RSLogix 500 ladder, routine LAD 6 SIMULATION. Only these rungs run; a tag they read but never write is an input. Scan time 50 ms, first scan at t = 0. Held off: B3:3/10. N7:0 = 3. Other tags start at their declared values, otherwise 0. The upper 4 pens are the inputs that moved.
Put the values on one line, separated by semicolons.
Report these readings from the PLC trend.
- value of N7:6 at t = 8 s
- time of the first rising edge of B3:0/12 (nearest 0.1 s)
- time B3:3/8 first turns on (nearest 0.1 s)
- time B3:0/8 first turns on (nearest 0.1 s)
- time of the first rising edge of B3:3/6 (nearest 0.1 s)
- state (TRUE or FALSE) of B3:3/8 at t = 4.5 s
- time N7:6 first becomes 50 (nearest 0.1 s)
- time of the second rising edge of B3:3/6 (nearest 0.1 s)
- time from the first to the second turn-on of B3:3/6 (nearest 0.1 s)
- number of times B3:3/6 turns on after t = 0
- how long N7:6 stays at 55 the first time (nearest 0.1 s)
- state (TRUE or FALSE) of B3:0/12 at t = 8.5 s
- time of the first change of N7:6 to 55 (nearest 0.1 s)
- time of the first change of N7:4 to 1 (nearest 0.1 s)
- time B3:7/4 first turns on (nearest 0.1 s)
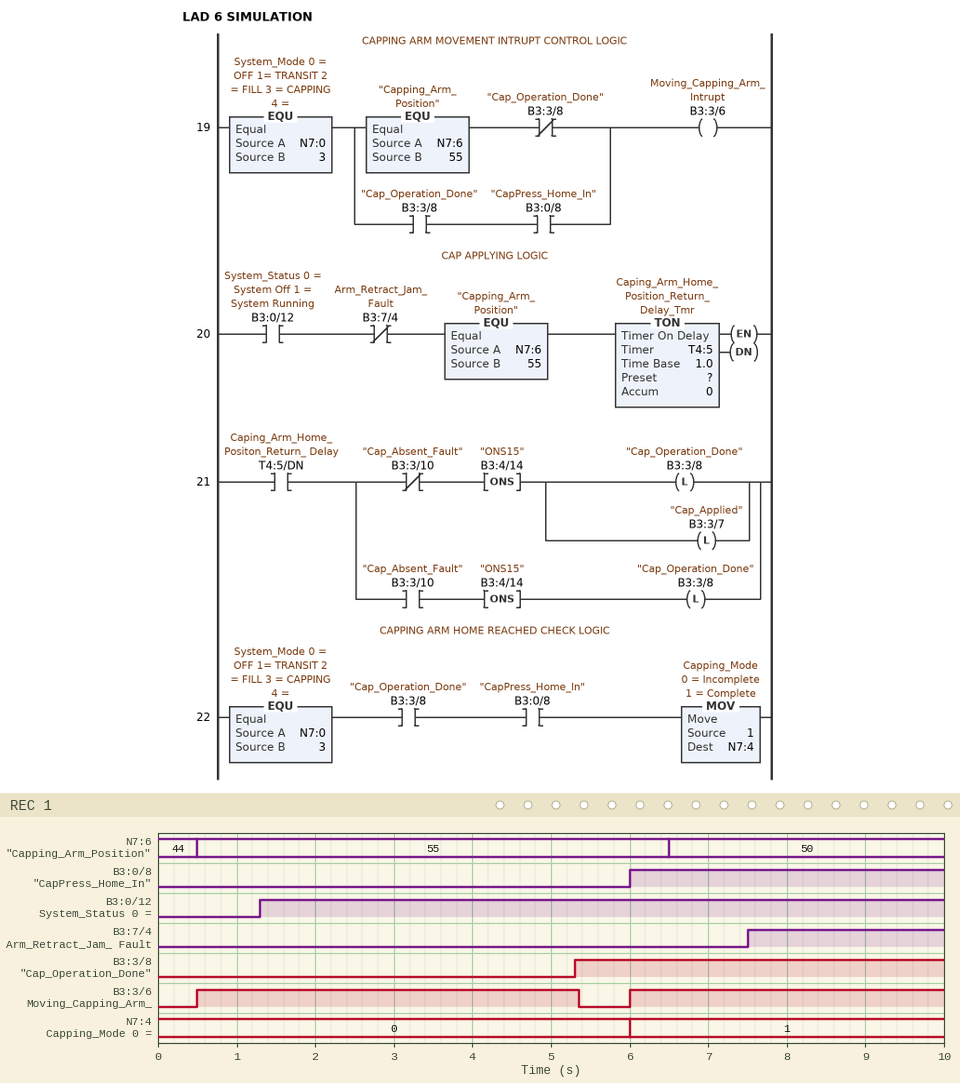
50; 1.3 s; 5.3 s; 6.0 s; 0.5 s; FALSE; 6.5 s; 6.0 s; 5.5 s; 2; 6.0 s; TRUE; 0.5 s; 6.0 s; 7.5 s
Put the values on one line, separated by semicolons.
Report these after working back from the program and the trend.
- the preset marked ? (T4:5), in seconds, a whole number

4 s
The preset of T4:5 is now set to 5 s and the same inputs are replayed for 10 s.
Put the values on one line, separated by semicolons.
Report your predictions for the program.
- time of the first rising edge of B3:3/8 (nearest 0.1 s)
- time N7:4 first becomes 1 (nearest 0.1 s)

6.3 s; 6.3 s
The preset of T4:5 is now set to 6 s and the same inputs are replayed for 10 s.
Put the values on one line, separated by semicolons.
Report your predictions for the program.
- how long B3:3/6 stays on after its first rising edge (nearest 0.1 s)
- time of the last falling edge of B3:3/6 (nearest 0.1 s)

6.0 s; 6.5 s
